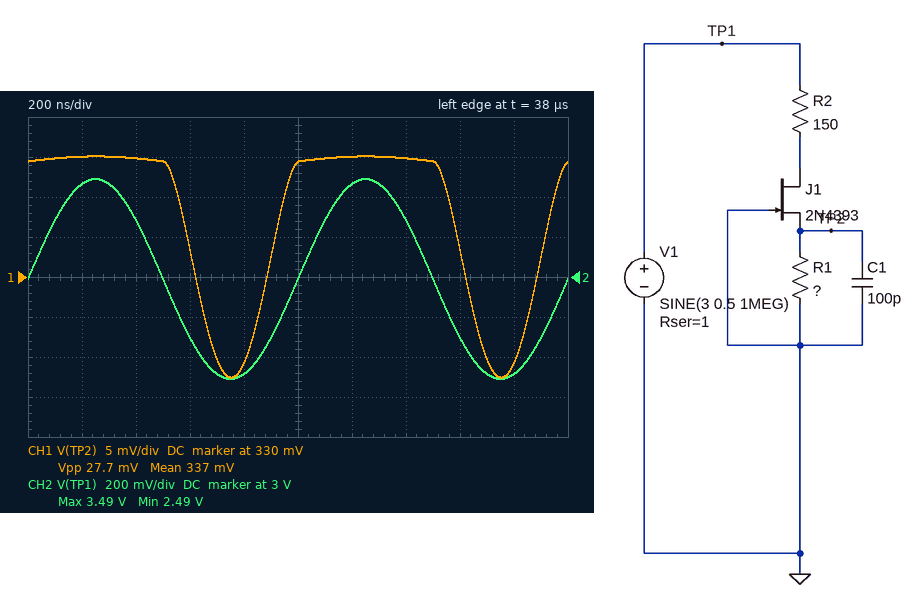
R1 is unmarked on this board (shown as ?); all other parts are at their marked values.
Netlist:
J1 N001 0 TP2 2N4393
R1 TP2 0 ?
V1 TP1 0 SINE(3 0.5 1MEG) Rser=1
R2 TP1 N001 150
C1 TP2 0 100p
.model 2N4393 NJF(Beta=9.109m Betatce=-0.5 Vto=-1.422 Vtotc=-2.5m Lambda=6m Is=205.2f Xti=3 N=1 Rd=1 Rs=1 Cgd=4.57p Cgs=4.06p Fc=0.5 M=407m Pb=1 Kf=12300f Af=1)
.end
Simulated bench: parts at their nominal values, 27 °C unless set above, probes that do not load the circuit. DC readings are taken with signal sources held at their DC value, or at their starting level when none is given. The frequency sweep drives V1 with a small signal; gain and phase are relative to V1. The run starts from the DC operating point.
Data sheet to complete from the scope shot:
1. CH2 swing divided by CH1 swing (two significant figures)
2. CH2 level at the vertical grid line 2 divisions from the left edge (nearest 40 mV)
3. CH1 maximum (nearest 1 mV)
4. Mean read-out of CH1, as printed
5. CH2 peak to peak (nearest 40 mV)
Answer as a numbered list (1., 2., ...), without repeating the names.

1. 36
2. 3.28 V
3. 345 mV
4. 337 mV
5. 1.00 V
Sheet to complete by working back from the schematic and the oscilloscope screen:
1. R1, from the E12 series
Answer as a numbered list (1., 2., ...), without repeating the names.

1. 33 Ω
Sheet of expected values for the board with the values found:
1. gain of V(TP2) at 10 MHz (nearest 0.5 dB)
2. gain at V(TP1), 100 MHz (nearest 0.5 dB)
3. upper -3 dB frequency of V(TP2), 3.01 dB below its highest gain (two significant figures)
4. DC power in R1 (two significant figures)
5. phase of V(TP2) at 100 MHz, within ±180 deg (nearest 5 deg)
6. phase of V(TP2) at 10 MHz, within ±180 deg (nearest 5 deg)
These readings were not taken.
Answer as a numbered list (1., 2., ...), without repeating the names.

1. -47.5 dB
2. 0 dB
3. 72 MHz
4. 3.6 mW
5. -70 deg
6. -10 deg
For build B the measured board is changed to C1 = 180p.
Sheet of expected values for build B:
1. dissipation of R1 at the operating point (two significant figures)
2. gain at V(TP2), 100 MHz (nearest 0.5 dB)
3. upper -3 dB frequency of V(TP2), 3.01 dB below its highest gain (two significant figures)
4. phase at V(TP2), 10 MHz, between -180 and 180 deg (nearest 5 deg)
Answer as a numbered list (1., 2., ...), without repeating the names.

1. 3.6 mW
2. -56.0 dB
3. 42 MHz
4. -15 deg
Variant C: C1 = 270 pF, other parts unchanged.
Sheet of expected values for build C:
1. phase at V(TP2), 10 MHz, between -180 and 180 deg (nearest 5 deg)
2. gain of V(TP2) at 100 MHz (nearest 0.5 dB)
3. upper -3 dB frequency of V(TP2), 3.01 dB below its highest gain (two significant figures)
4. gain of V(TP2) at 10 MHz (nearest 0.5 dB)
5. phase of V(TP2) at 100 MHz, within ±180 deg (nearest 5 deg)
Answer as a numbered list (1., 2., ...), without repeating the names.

1. -20 deg
2. -59.0 dB
3. 28 MHz
4. -48.0 dB
5. -90 deg
